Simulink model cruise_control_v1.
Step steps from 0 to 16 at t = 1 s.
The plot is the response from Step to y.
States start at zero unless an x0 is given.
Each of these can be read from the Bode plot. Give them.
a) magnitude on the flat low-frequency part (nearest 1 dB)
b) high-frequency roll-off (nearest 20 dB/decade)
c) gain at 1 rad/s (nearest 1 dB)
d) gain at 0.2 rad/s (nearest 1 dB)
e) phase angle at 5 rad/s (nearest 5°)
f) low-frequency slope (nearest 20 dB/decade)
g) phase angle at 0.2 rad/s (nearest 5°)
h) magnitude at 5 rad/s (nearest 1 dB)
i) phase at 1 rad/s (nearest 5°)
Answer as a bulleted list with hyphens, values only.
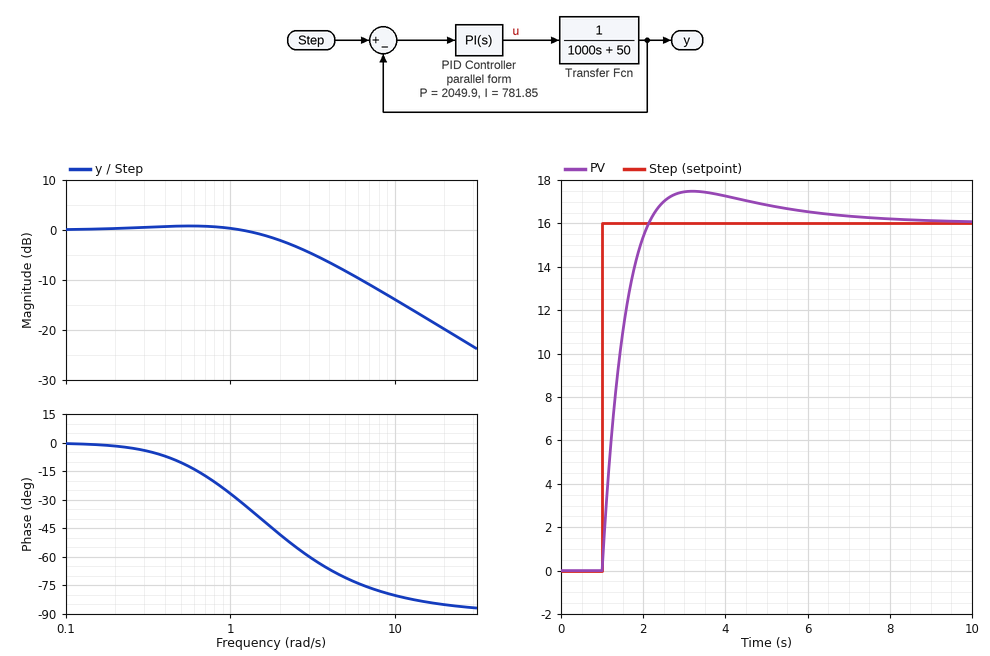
- 0 dB
- -20 dB/decade
- 0 dB
- 0 dB
- -70°
- 0 dB/decade
- 0°
- -8 dB
- -25°
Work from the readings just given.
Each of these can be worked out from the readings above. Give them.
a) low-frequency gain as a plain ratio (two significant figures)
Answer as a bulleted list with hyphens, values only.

- 1.0
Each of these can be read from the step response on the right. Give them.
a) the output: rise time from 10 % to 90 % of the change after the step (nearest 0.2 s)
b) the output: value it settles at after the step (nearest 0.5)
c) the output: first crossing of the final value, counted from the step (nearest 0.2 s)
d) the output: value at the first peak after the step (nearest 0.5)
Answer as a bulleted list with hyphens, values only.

- 0.8 s
- 16.0
- 1.2 s
- 17.5
